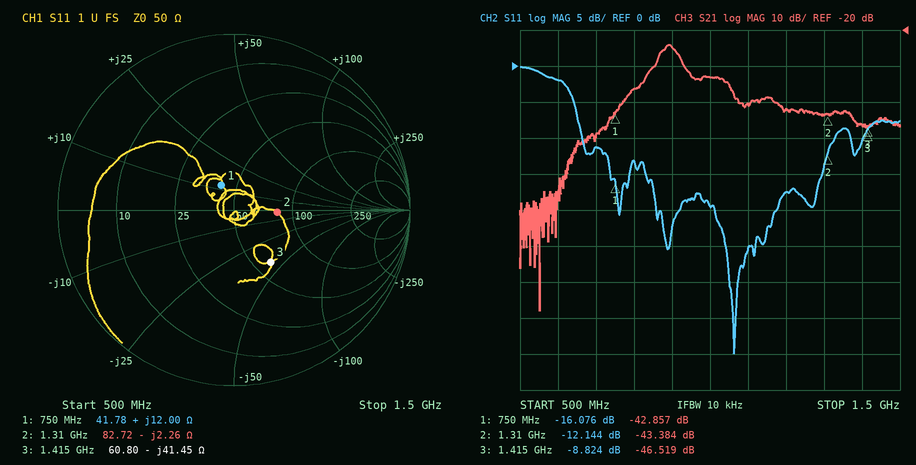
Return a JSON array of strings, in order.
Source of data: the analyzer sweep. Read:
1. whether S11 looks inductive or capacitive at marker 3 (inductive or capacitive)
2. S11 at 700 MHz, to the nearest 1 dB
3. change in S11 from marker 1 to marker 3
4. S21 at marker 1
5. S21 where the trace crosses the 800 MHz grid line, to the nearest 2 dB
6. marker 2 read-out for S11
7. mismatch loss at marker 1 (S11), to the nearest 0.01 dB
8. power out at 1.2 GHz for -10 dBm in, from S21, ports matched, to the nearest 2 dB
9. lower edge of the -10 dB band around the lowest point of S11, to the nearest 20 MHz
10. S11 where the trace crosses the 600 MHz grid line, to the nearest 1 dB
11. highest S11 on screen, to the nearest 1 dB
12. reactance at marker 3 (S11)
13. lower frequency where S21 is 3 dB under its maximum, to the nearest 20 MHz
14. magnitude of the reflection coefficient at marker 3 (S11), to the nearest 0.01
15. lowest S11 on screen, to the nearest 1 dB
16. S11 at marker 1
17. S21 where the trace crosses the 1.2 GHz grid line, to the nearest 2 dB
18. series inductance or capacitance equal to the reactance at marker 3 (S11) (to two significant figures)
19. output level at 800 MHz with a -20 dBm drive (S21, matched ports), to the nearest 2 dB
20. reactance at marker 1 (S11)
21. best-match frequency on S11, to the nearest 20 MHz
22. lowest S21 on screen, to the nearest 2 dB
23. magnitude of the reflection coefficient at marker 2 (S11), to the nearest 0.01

["capacitive", "-11 dB", "7.252 dB", "-42.857 dB", "-36 dB", "-12.144 dB", "0.11 dB", "-52 dBm", "660 MHz", "-2 dB", "0 dB", "-41.45 Ω", "860 MHz", "0.36", "-40 dB", "-16.076 dB", "-42 dB", "2.7 pF", "-56 dBm", "+12.00 Ω", "1.06 GHz", "-98 dB", "0.25"]
